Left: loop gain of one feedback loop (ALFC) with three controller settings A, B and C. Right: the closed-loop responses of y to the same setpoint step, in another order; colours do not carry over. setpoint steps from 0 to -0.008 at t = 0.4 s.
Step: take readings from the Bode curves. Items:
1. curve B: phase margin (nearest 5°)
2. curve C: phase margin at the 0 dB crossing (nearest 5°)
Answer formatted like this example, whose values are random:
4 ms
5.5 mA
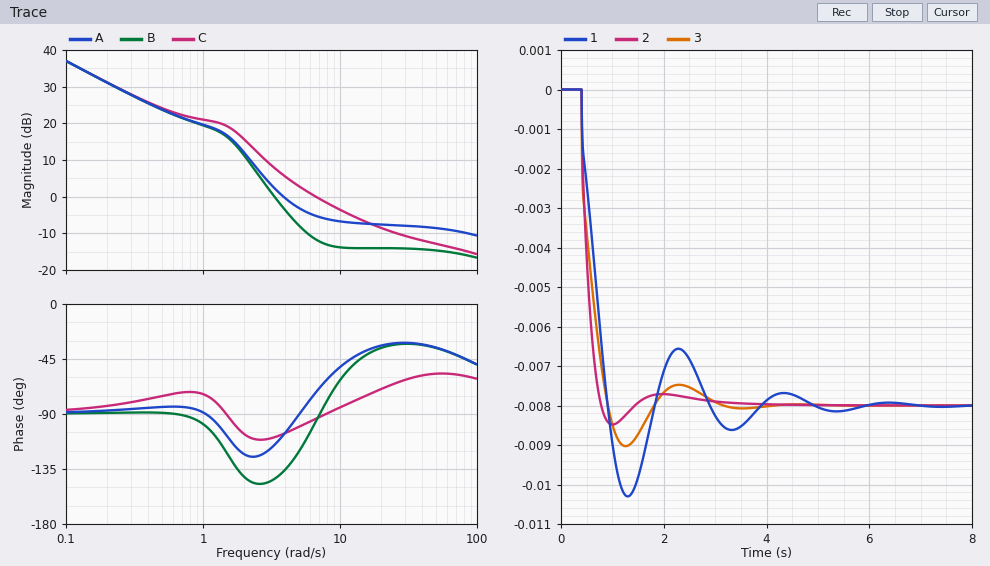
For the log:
35°
85°
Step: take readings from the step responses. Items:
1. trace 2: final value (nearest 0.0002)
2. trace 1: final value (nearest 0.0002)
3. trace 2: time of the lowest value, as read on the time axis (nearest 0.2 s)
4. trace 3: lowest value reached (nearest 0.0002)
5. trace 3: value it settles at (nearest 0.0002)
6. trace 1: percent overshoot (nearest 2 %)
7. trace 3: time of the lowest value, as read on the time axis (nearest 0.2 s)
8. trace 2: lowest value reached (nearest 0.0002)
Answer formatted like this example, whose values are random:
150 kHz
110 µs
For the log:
-0.0080
-0.0080
1.0 s
-0.0090
-0.0080
28 %
1.2 s
-0.0084
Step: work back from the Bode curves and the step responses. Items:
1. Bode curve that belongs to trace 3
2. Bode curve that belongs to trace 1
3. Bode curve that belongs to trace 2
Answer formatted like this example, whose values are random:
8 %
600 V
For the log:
A
B
C
